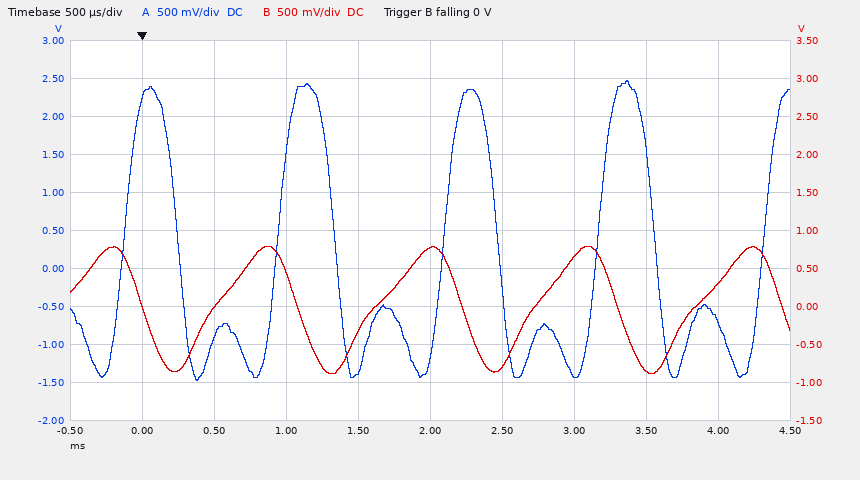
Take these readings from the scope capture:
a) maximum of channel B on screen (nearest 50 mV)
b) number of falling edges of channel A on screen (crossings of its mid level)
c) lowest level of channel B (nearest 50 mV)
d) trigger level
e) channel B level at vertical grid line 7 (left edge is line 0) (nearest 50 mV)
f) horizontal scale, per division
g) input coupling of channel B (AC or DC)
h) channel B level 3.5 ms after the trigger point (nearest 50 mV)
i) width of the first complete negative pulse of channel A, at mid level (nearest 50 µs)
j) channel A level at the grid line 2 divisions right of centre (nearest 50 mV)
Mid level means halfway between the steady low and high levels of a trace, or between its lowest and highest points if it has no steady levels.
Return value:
800 mV
4
-900 mV
0 V
650 mV
500 µs
DC
-850 mV
700 µs
-1.40 V
